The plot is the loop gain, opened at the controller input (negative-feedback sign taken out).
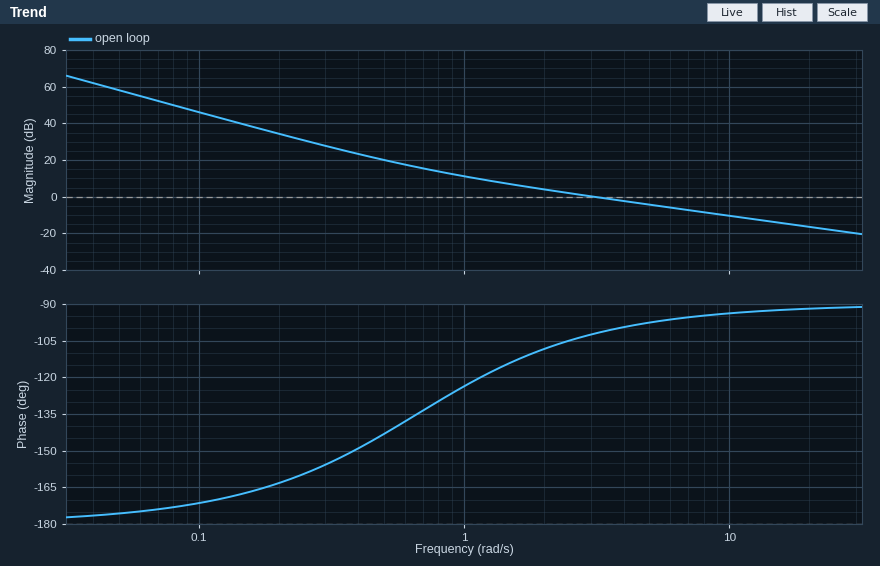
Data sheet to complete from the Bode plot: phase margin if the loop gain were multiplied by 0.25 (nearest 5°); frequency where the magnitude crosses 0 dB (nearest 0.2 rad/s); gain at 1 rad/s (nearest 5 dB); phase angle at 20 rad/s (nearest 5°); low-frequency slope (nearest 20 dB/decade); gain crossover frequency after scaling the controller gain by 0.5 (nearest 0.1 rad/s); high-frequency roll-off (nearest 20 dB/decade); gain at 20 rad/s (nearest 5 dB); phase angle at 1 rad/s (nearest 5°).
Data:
55°
3.0 rad/s
10 dB
-90°
-40 dB/decade
1.6 rad/s
-20 dB/decade
-15 dB
-125°
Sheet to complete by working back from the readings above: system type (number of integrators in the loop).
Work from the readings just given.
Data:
2
